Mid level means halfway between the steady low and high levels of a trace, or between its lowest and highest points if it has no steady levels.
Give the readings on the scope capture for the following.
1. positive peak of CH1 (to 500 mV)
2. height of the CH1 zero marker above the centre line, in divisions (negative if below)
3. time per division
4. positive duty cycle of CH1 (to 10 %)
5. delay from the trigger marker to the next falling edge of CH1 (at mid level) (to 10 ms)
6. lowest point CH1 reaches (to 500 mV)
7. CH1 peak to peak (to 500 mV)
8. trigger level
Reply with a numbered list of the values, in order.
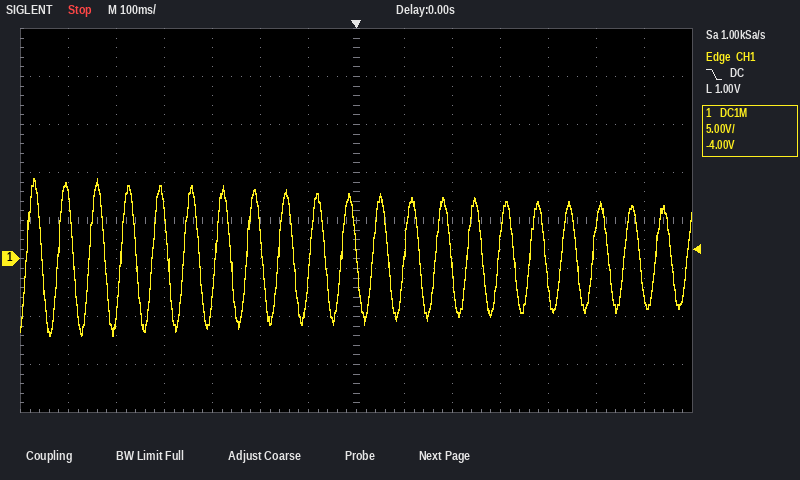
1. 8.5 V
2. -0.8 div
3. 100 ms
4. 50 %
5. 70 ms
6. -8.0 V
7. 16.5 V
8. 1.00 V
